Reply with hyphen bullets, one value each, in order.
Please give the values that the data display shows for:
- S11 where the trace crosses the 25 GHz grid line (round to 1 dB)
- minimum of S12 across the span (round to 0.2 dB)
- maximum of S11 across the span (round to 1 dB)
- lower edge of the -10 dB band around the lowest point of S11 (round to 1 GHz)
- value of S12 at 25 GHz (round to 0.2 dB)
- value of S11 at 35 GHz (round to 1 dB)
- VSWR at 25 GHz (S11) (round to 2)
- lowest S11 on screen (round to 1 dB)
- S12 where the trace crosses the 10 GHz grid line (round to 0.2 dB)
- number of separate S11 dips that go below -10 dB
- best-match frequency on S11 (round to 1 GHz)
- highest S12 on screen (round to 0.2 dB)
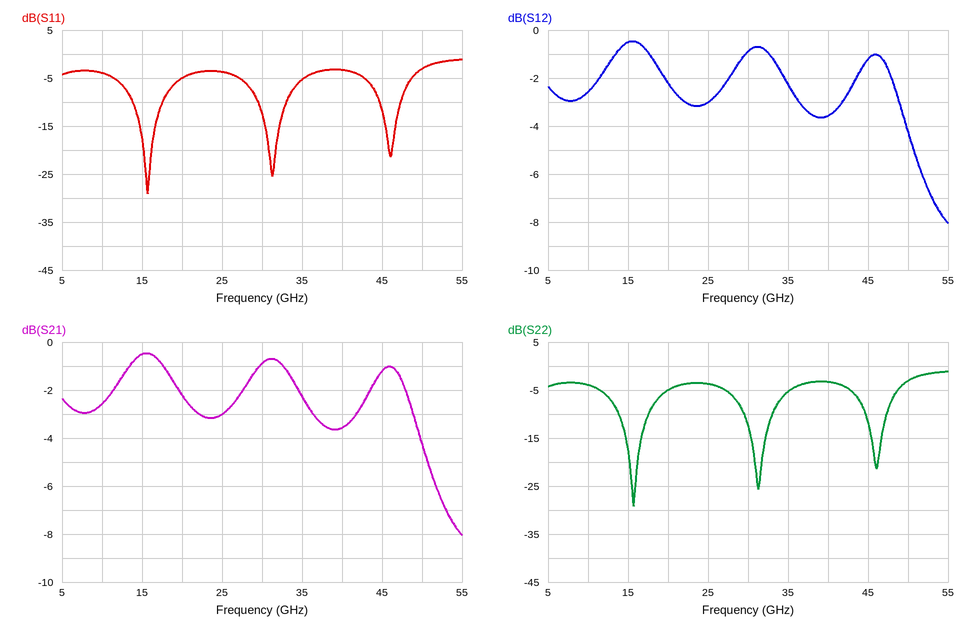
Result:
- -4 dB
- -8.0 dB
- -1 dB
- 14 GHz
- -3.0 dB
- -5 dB
- 4
- -29 dB
- -2.6 dB
- 3
- 16 GHz
- -0.4 dB
